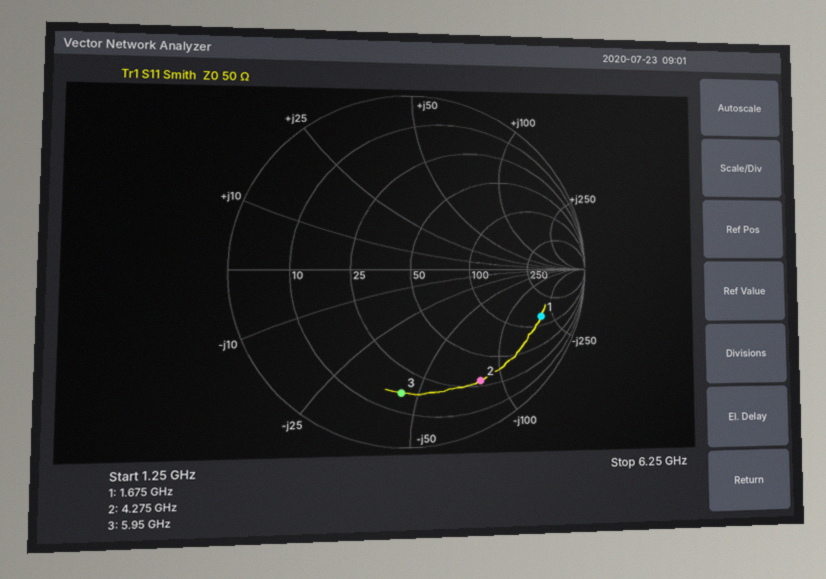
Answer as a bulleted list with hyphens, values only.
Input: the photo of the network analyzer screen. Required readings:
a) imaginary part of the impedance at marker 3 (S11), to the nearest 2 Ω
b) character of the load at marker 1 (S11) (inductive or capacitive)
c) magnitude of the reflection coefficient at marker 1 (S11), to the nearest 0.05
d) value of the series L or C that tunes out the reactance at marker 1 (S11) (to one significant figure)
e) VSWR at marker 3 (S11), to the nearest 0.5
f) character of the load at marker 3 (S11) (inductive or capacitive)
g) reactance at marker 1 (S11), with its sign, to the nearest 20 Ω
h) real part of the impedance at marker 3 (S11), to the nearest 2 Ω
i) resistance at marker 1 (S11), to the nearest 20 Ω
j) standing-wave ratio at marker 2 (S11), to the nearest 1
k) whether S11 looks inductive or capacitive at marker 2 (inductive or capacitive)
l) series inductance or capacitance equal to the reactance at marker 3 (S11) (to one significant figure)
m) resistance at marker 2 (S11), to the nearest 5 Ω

- -44 Ω
- capacitive
- 0.80
- 20 nH
- 5.5
- capacitive
- -200 Ω
- 16 Ω
- 140 Ω
- 7
- capacitive
- 600 fF
- 30 Ω
